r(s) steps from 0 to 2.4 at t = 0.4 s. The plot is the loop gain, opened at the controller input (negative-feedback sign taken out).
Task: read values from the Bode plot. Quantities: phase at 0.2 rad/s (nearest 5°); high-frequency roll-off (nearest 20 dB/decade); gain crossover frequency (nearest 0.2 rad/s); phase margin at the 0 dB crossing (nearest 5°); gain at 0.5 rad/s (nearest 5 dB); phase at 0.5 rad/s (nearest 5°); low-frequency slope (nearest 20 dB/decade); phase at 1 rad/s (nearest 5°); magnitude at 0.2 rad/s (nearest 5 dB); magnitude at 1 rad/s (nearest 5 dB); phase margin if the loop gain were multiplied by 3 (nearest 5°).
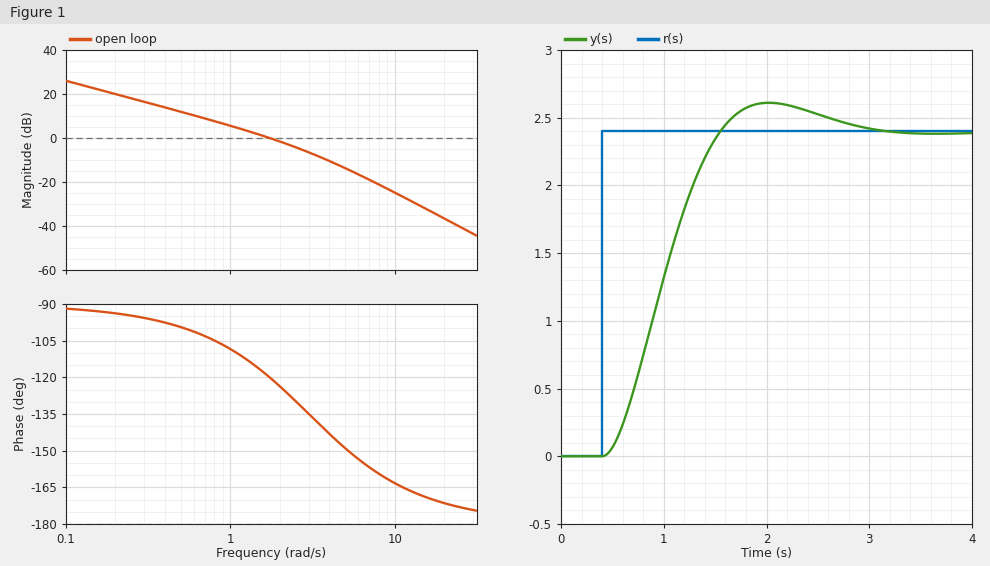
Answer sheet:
-95°
-40 dB/decade
1.8 rad/s
60°
10 dB
-100°
-20 dB/decade
-110°
20 dB
5 dB
40°
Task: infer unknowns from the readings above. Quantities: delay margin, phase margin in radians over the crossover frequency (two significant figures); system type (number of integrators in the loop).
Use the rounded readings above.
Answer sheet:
0.58 s
1
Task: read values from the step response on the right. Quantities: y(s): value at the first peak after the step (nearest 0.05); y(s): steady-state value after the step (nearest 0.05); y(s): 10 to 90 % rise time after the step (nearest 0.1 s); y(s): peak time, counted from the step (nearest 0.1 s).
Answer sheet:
2.60
2.40
0.8 s
1.6 s
